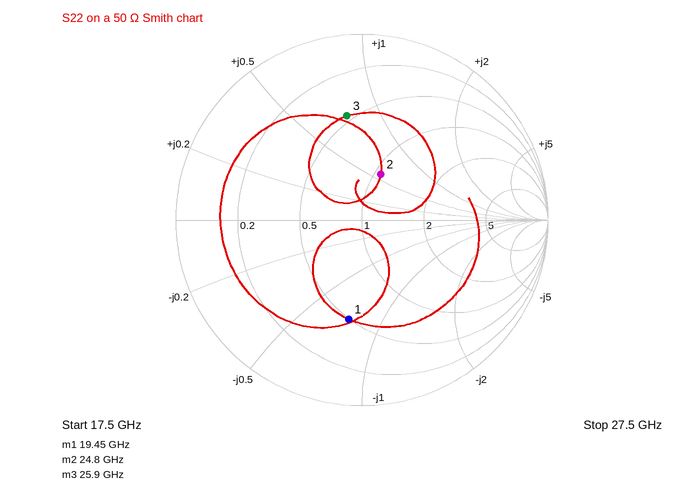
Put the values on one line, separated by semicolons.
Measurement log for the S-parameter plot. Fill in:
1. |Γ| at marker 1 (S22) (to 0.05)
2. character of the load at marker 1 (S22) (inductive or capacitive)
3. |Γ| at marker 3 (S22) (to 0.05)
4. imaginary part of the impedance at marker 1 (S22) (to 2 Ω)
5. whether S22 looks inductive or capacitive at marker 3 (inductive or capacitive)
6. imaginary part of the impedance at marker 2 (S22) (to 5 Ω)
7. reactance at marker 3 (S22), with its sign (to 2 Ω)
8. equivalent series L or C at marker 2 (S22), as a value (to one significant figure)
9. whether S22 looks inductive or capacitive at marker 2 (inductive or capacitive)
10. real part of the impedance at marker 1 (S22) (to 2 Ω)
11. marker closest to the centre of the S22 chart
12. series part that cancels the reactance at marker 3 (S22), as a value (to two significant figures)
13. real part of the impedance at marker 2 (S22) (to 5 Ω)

0.55; capacitive; 0.55; -38 Ω; inductive; +30 Ω; +38 Ω; 200 pH; inductive; 24 Ω; marker 2; 160 fF; 55 Ω
